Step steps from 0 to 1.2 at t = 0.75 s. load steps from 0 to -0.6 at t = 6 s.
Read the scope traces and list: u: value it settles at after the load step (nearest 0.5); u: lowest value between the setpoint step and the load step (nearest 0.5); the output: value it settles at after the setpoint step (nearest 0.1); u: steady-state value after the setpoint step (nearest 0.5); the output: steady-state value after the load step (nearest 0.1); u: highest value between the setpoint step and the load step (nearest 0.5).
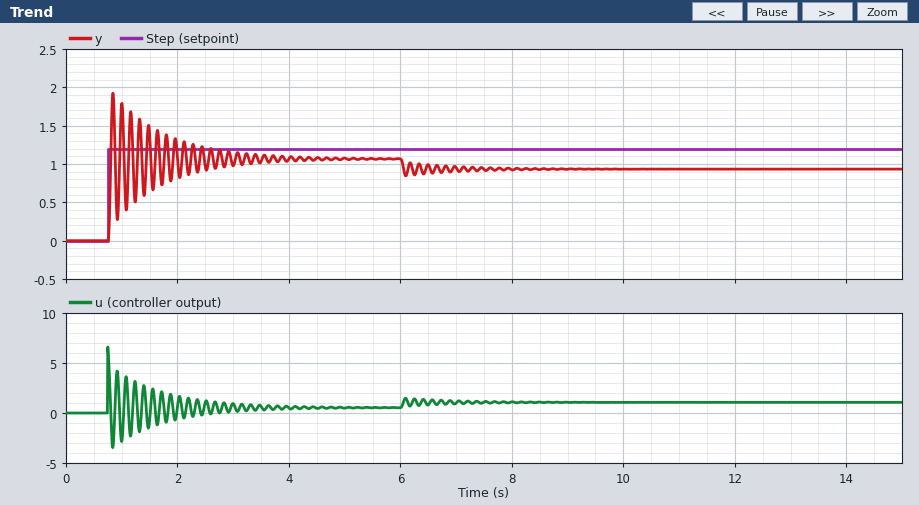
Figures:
1.0
-3.5
1.1
0.5
0.9
6.5
